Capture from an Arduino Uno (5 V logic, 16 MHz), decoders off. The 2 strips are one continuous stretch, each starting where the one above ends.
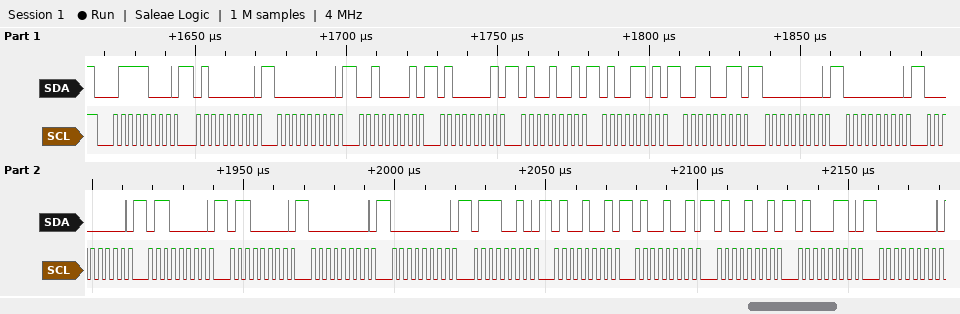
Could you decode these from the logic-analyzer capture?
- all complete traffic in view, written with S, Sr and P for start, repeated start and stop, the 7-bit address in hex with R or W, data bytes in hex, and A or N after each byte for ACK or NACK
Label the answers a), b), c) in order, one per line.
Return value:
a) S 3CW A 40 A 00 A 21 A 41 A 49 A 4D A 33 A 00 A 00 A 00 A 60 A 60 A 00 A 00 A 72 A 49 A 49 A 49 A 46 A 00 A
